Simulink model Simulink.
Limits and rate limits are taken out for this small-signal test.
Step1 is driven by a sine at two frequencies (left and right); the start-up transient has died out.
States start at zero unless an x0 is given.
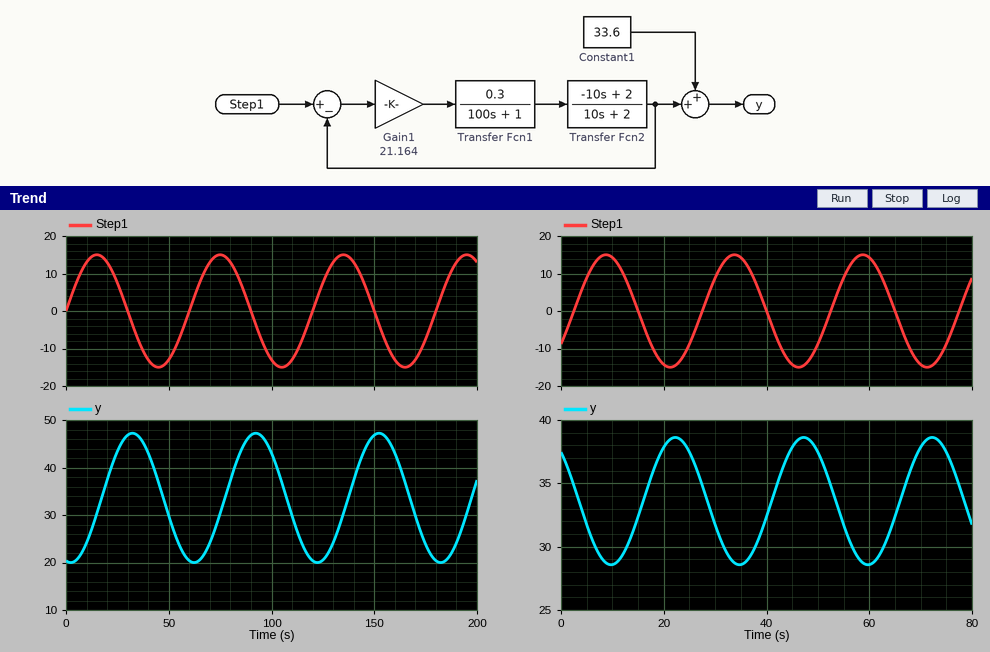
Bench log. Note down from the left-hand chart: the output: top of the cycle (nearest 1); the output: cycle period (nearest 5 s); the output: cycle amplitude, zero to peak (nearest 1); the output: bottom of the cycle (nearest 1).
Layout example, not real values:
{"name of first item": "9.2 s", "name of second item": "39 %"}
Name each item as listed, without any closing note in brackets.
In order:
{"the output: top of the cycle": "47", "the output: cycle period": "60 s", "the output: cycle amplitude, zero to peak": "14", "the output: bottom of the cycle": "20"}
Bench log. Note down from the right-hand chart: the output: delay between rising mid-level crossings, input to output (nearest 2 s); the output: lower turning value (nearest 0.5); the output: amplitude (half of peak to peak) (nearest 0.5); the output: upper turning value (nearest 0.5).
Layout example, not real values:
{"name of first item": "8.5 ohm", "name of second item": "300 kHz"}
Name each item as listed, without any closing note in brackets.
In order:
{"the output: delay between rising mid-level crossings, input to output": "14 s", "the output: lower turning value": "28.5", "the output: amplitude (half of peak to peak)": "5.0", "the output: upper turning value": "38.5"}
